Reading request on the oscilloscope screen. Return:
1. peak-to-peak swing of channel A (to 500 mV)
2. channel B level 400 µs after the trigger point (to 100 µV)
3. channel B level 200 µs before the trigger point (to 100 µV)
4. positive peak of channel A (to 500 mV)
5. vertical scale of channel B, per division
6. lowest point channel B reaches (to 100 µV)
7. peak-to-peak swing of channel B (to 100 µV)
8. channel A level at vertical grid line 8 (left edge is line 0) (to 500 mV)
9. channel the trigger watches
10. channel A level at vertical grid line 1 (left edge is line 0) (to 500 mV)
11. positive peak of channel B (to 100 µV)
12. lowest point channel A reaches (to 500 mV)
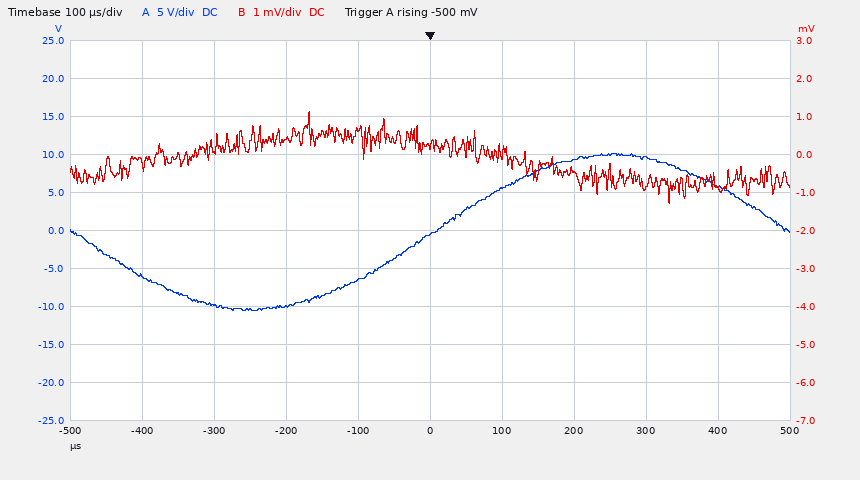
20.5 V
-900 µV
400 µV
10.0 V
1 mV
-1.3 mV
2.4 mV
9.5 V
channel A
-6.0 V
1.1 mV
-10.5 V
